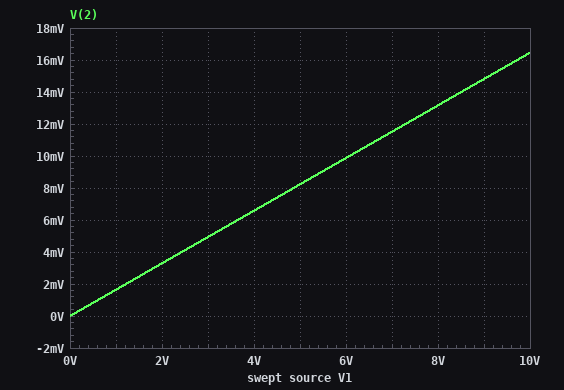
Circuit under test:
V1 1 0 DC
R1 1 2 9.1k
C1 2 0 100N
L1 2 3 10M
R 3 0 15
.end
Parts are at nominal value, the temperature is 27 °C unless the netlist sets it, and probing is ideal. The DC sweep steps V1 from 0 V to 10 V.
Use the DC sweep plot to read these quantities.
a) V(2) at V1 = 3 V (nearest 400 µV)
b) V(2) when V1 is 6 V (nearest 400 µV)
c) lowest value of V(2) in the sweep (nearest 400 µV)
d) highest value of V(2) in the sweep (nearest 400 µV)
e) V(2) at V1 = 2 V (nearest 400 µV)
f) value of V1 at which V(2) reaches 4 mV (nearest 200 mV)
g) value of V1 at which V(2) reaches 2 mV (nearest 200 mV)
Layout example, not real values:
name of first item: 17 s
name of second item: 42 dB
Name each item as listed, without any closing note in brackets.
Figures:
V(2) at V1 = 3 V: 4.8 mV
V(2) when V1 is 6 V: 10.0 mV
lowest value of V(2) in the sweep: 0 V
highest value of V(2) in the sweep: 16.4 mV
V(2) at V1 = 2 V: 3.2 mV
value of V1 at which V(2) reaches 4 mV: 2.4 V
value of V1 at which V(2) reaches 2 mV: 1.2 V
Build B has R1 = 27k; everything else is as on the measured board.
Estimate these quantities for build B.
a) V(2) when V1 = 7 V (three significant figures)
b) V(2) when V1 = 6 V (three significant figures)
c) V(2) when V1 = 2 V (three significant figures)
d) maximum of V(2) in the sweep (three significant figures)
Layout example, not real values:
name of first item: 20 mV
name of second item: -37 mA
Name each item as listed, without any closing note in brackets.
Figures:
V(2) when V1 = 7 V: 3.89 mV
V(2) when V1 = 6 V: 3.33 mV
V(2) when V1 = 2 V: 1.11 mV
maximum of V(2) in the sweep: 5.55 mV
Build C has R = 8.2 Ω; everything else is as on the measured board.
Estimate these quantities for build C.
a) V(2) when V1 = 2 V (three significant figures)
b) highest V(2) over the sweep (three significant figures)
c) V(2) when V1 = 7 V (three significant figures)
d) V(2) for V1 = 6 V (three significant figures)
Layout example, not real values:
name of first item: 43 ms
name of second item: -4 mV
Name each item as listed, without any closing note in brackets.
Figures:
V(2) when V1 = 2 V: 1.80 mV
highest V(2) over the sweep: 9.00 mV
V(2) when V1 = 7 V: 6.30 mV
V(2) for V1 = 6 V: 5.40 mV
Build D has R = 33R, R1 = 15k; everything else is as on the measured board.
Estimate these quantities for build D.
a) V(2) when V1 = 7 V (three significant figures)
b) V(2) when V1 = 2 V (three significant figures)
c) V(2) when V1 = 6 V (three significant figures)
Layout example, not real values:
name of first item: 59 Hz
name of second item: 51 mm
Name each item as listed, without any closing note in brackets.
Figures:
V(2) when V1 = 7 V: 15.4 mV
V(2) when V1 = 2 V: 4.39 mV
V(2) when V1 = 6 V: 13.2 mV
